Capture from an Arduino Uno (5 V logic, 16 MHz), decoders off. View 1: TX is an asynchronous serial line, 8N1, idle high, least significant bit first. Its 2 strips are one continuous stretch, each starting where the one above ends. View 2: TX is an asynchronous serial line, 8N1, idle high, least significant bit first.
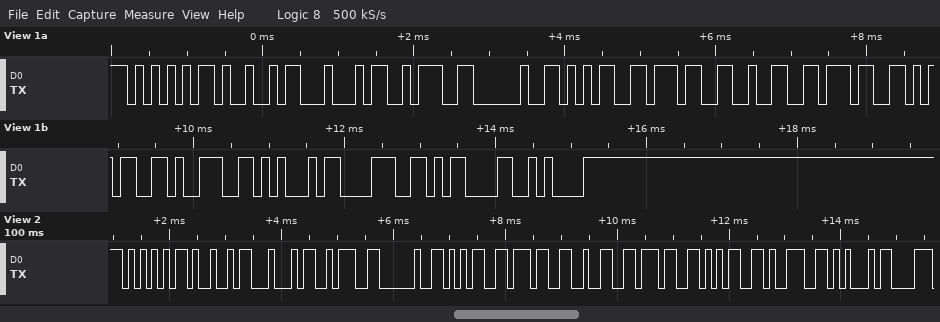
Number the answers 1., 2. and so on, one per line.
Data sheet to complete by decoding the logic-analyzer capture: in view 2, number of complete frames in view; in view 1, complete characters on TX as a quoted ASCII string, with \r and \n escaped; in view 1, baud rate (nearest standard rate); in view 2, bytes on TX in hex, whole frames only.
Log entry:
1. 12
2. "UID: 572759E8\r\n"
3. 9600 baud
4. 0x55 0x49 0x44 0x3A 0x20 0x35 0x37 0x32 0x37 0x35 0x39 0x45
